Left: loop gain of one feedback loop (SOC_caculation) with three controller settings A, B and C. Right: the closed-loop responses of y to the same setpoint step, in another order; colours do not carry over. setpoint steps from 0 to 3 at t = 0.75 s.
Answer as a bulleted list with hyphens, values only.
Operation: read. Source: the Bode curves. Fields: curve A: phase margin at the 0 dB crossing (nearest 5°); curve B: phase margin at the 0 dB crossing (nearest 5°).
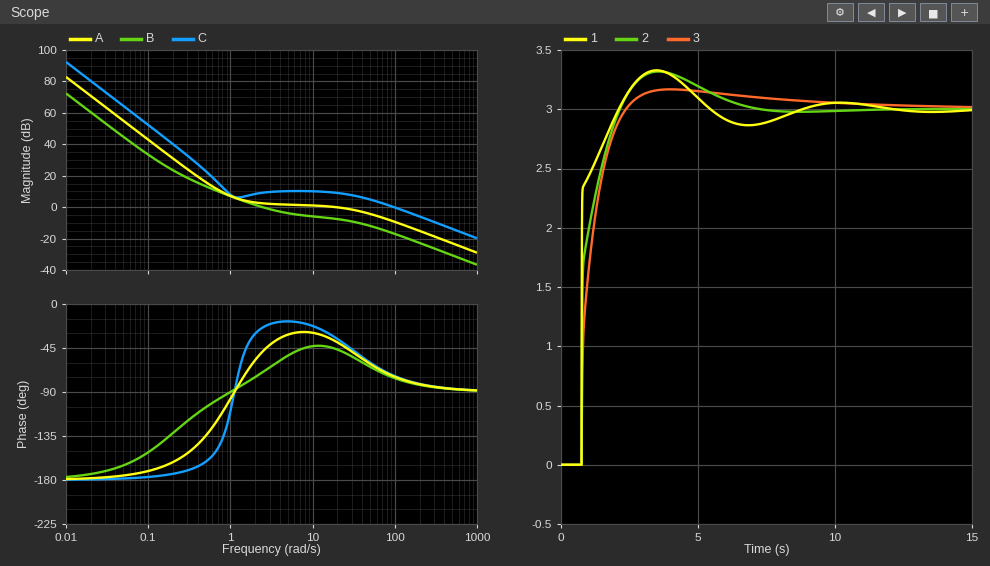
- 140°
- 110°
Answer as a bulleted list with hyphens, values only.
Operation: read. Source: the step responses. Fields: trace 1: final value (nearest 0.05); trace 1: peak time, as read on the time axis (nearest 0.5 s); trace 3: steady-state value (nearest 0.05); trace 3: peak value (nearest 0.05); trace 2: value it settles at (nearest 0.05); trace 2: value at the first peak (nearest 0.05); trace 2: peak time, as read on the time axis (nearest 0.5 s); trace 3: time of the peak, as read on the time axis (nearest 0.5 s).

- 3.00
- 3.5 s
- 3.00
- 3.15
- 3.00
- 3.30
- 3.5 s
- 4.0 s
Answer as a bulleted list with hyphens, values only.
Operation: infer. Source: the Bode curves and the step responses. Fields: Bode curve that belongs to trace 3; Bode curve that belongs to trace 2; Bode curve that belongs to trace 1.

- B
- A
- C
